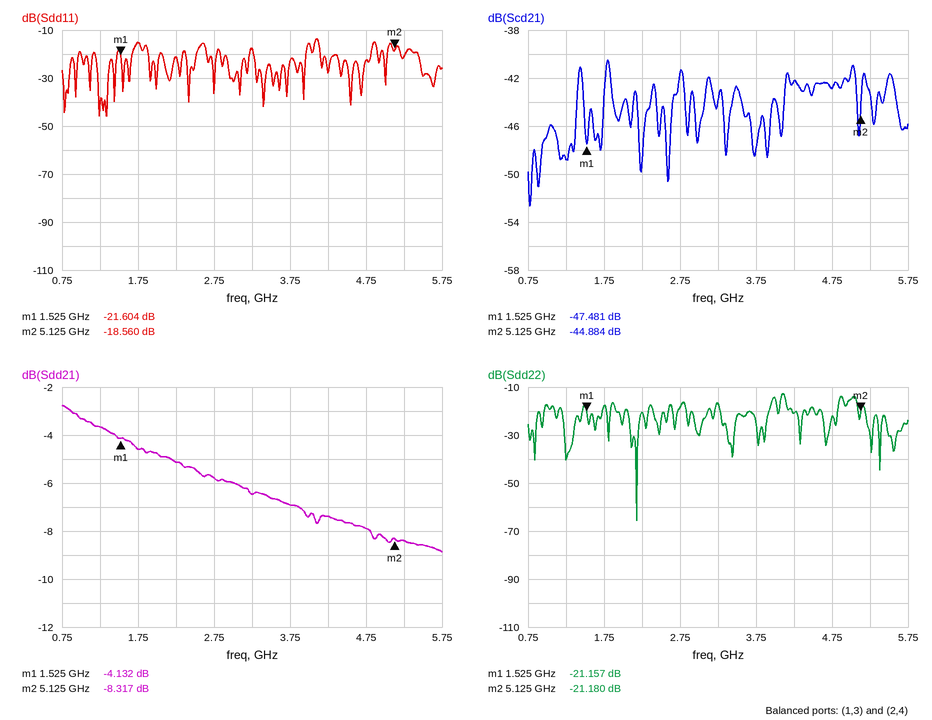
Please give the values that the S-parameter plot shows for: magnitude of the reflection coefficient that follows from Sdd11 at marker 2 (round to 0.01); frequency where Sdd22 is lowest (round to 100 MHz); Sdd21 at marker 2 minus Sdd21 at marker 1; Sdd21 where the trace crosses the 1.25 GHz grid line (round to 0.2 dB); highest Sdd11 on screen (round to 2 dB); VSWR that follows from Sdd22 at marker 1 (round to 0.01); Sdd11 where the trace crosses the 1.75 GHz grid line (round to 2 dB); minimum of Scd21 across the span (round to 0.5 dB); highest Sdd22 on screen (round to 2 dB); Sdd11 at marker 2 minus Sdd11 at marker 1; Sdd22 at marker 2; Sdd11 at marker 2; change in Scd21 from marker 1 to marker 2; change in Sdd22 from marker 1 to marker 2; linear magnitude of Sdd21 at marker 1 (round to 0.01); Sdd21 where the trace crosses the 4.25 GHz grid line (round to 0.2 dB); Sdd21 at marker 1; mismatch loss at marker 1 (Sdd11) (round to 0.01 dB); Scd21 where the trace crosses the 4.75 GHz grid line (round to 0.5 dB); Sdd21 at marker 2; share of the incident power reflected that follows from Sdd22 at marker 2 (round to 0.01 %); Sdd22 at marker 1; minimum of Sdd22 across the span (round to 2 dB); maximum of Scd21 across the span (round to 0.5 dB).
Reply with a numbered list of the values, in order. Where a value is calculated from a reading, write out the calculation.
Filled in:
1. 10^(-18.56/20) ≈ 0.12
2. 2.2 GHz
3. -8.317 − (-4.132) = -4.185 dB
4. -3.6 dB
5. -14 dB
6. (1 + 0.0875)/(1 − 0.0875) ≈ 1.19
7. -16 dB
8. -52.5 dB
9. -12 dB
10. -18.56 − (-21.604) = 3.044 dB
11. -21.180 dB
12. -18.560 dB
13. -44.884 − (-47.481) = 2.597 dB
14. -21.18 − (-21.157) = -0.023 dB
15. 10^(-4.132/20) ≈ 0.62
16. -7.4 dB
17. -4.132 dB
18. −10 log10(1 − 10^(-21.604/10)) ≈ 0.03 dB
19. -43.0 dB
20. -8.317 dB
21. 10^(-21.18/10) ≈ 0.76 %
22. -21.157 dB
23. -66 dB
24. -40.5 dB
